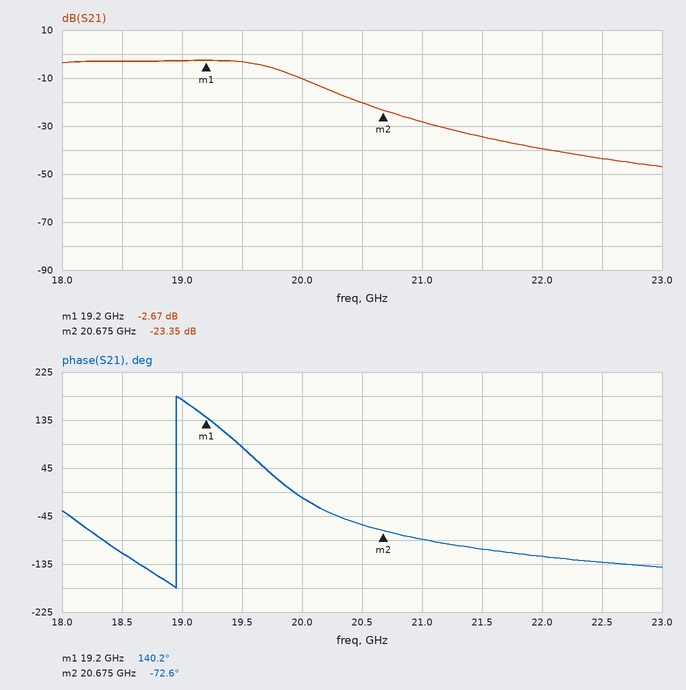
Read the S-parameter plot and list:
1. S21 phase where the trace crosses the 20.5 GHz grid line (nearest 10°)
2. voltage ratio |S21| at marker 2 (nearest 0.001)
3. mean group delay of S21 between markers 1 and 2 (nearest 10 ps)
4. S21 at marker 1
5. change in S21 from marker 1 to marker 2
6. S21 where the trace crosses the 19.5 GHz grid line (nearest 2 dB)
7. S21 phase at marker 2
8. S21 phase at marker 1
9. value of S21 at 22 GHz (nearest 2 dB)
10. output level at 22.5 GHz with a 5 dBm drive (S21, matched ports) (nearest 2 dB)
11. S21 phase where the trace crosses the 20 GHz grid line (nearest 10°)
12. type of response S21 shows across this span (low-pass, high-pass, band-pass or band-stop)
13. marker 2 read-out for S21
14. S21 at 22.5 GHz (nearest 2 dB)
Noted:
-60°
0.068
400 ps
-2.67 dB
-20.68 dB
-4 dB
-72.6°
140.2°
-40 dB
-38 dBm
-10°
low-pass
-23.35 dB
-44 dB
